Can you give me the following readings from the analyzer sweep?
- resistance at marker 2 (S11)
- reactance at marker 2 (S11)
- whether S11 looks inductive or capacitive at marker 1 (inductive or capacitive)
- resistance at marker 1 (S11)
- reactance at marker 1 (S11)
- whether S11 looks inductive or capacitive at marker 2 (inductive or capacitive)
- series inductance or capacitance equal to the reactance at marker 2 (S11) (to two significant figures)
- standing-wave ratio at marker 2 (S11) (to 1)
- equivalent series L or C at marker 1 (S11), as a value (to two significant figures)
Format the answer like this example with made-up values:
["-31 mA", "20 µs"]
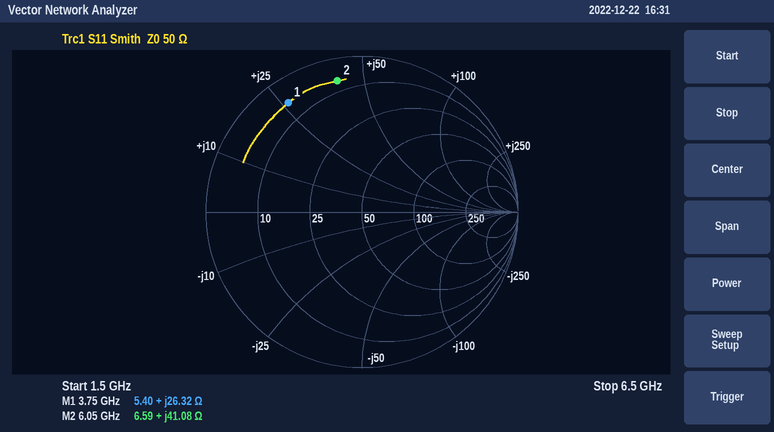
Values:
["6.59 Ω", "+41.08 Ω", "inductive", "5.40 Ω", "+26.32 Ω", "inductive", "1.1 nH", "13", "1.1 nH"]
